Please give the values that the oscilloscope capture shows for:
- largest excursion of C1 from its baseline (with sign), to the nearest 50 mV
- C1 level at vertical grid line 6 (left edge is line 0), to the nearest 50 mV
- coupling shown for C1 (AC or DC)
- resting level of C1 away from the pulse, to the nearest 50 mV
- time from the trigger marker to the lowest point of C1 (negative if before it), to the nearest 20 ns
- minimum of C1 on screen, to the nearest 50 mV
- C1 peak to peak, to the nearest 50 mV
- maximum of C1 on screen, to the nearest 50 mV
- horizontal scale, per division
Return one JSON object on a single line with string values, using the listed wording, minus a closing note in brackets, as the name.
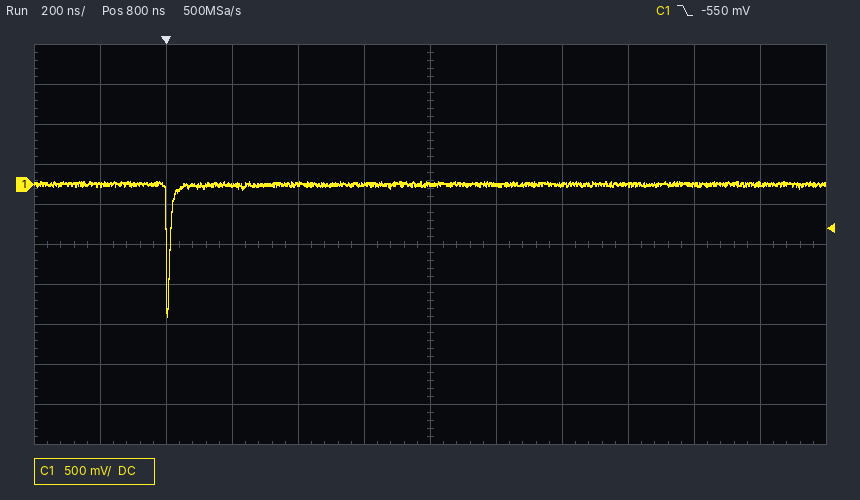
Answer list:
{"largest excursion of C1 from its baseline (with sign), to the nearest 50 mV": "-1.65 V", "C1 level at vertical grid line 6 (left edge is line 0), to the nearest 50 mV": "0 mV", "coupling shown for C1": "DC", "resting level of C1 away from the pulse, to the nearest 50 mV": "0 mV", "time from the trigger marker to the lowest point of C1 (negative if before it), to the nearest 20 ns": "0 ns", "minimum of C1 on screen, to the nearest 50 mV": "-1.65 V", "C1 peak to peak, to the nearest 50 mV": "1.70 V", "maximum of C1 on screen, to the nearest 50 mV": "50 mV", "horizontal scale, per division": "200 ns"}
